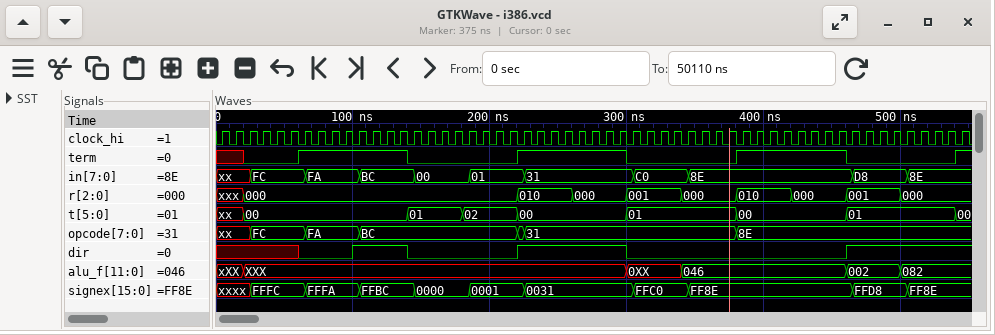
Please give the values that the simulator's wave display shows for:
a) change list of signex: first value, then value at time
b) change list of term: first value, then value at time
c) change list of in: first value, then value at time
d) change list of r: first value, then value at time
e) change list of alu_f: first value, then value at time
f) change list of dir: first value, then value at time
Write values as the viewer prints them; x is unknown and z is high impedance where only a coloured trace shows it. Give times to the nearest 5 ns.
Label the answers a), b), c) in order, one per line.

a) xxxx, FFFC at 25 ns, FFFA at 65 ns, FFBC at 105 ns, 0000 at 145 ns, 0001 at 185 ns, 0031 at 225 ns, FFC0 at 305 ns, FF8E at 345 ns, FFD8 at 465 ns, FF8E at 505 ns
b) x, 0 at 20 ns, 1 at 60 ns, 0 at 140 ns, 1 at 220 ns, 0 at 300 ns, 1 at 380 ns, 0 at 460 ns, 1 at 540 ns
c) xx, FC at 25 ns, FA at 65 ns, BC at 105 ns, 00 at 145 ns, 01 at 185 ns, 31 at 225 ns, C0 at 305 ns, 8E at 345 ns, D8 at 465 ns, 8E at 505 ns
d) xxx, 000 at 20 ns, 010 at 220 ns, 000 at 260 ns, 001 at 300 ns, 000 at 340 ns, 010 at 380 ns, 000 at 420 ns, 001 at 460 ns, 000 at 500 ns
e) xXX, XXX at 20 ns, 0XX at 300 ns, 046 at 340 ns, 002 at 460 ns, 082 at 500 ns
f) x, 0 at 60 ns, 1 at 100 ns, 0 at 140 ns, 1 at 220 ns, 0 at 300 ns, 1 at 460 ns
